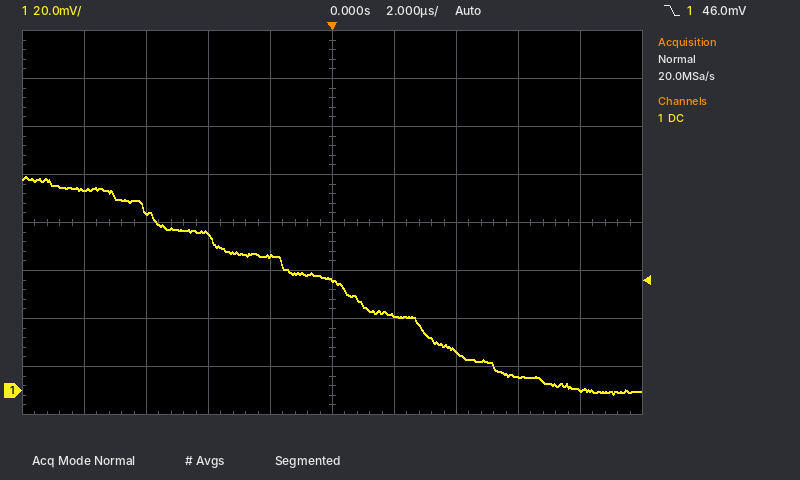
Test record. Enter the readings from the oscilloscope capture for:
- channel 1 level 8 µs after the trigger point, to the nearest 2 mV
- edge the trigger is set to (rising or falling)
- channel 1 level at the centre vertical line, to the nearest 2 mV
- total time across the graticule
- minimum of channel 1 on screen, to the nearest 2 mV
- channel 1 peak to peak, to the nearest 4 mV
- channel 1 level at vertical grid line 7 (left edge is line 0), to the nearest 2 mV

0 mV
falling
46 mV
20 µs
-2 mV
92 mV
16 mV
